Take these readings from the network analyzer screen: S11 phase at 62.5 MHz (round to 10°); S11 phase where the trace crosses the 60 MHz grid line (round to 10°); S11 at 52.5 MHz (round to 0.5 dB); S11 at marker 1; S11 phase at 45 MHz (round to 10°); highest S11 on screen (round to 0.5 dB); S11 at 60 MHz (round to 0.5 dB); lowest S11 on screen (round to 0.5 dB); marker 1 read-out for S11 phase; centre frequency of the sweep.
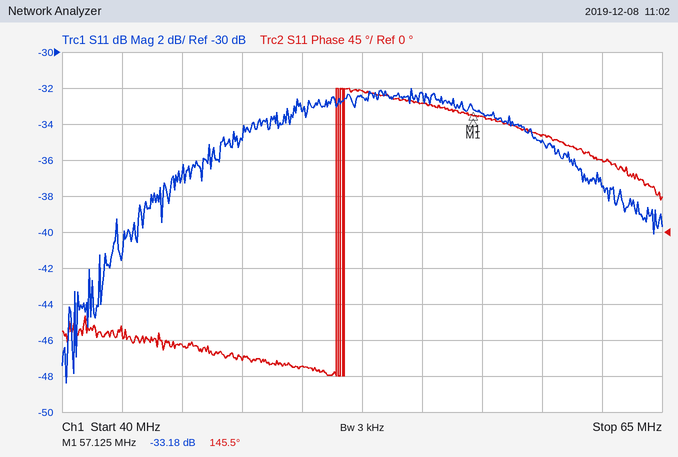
90°
120°
-32.5 dB
-33.18 dB
-140°
-32.0 dB
-35.0 dB
-48.5 dB
145.5°
52.5 MHz
